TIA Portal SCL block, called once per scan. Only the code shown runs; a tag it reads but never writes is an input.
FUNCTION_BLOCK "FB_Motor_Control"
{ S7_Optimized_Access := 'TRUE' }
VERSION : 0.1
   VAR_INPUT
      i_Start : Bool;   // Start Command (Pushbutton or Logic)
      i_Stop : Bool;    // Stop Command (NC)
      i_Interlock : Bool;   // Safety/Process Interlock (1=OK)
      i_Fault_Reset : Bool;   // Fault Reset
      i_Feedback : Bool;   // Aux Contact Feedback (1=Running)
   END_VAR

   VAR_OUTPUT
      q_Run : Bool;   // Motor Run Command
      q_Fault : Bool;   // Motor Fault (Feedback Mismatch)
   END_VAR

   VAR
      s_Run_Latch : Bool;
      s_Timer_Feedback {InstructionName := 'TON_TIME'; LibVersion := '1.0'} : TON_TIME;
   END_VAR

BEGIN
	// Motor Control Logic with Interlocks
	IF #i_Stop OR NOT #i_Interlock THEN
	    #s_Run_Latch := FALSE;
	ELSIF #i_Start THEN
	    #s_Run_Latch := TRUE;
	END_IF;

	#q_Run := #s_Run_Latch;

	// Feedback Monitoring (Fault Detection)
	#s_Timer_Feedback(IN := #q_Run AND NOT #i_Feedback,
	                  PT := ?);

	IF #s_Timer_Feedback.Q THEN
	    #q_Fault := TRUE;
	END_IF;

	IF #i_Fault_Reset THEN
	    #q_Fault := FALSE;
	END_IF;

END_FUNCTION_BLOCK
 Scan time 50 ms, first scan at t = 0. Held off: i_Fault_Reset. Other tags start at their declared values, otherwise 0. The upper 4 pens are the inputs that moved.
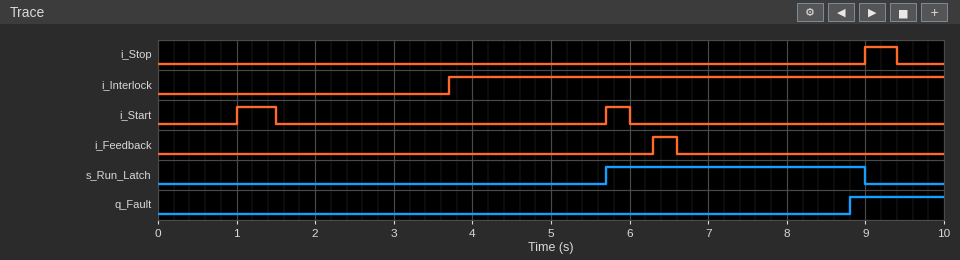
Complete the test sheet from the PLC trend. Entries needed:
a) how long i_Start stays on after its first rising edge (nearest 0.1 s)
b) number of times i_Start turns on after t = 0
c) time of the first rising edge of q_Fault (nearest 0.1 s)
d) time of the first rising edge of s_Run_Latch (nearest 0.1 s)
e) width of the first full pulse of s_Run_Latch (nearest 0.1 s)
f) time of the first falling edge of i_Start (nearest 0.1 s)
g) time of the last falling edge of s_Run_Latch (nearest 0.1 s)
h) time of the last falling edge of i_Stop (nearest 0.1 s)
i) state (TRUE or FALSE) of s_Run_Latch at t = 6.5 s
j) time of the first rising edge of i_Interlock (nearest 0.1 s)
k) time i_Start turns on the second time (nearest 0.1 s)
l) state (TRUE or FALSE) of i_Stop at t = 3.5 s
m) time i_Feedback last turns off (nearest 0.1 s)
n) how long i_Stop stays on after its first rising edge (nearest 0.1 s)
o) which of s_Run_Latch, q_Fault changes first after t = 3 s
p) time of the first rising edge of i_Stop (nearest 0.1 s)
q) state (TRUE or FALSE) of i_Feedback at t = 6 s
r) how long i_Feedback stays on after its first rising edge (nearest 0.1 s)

0.5 s
2
8.8 s
5.7 s
3.3 s
1.5 s
9.0 s
9.4 s
TRUE
3.7 s
5.7 s
FALSE
6.6 s
0.4 s
s_Run_Latch
9.0 s
FALSE
0.3 s
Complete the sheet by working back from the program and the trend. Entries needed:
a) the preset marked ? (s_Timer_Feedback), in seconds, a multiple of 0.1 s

2.2 s
